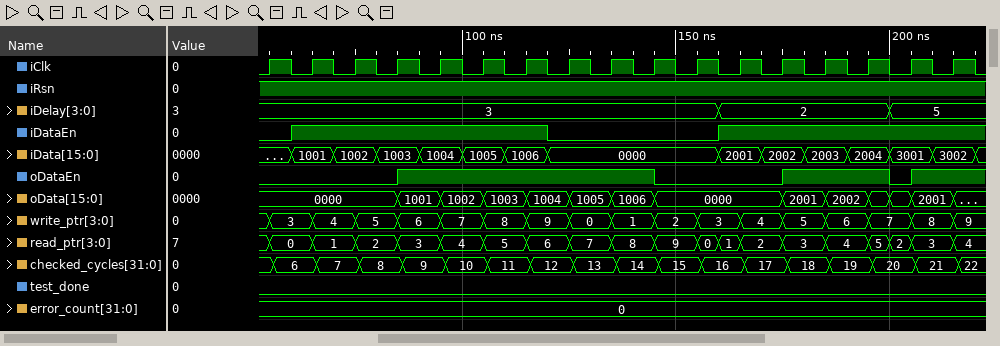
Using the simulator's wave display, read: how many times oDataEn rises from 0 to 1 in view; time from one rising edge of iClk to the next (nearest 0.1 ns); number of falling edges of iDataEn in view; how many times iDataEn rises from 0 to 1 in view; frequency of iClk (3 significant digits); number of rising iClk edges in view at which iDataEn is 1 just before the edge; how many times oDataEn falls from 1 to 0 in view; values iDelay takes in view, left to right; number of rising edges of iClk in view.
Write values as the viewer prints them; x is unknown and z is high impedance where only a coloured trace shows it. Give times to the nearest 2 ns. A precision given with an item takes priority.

3
10 ns
1
2
100 MHz
12
2
3, 2, 5
17
